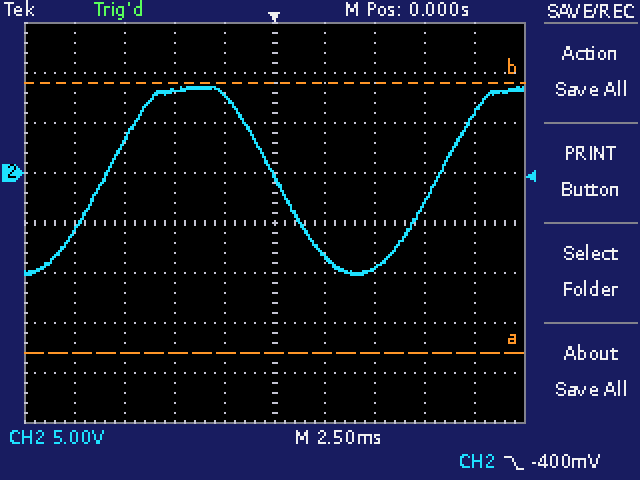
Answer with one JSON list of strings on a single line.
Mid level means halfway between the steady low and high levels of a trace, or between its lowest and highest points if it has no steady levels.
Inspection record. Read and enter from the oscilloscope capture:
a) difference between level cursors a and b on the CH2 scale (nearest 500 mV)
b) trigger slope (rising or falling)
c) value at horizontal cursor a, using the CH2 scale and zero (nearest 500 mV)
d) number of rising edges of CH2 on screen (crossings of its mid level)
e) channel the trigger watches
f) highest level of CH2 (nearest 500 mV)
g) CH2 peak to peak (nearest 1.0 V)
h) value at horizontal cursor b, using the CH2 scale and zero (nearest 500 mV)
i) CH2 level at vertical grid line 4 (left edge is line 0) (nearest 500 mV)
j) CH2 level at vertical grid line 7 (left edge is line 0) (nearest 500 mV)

["27.0 V", "falling", "-18.0 V", "2", "CH2", "8.5 V", "19.0 V", "9.0 V", "8.0 V", "-9.5 V"]
